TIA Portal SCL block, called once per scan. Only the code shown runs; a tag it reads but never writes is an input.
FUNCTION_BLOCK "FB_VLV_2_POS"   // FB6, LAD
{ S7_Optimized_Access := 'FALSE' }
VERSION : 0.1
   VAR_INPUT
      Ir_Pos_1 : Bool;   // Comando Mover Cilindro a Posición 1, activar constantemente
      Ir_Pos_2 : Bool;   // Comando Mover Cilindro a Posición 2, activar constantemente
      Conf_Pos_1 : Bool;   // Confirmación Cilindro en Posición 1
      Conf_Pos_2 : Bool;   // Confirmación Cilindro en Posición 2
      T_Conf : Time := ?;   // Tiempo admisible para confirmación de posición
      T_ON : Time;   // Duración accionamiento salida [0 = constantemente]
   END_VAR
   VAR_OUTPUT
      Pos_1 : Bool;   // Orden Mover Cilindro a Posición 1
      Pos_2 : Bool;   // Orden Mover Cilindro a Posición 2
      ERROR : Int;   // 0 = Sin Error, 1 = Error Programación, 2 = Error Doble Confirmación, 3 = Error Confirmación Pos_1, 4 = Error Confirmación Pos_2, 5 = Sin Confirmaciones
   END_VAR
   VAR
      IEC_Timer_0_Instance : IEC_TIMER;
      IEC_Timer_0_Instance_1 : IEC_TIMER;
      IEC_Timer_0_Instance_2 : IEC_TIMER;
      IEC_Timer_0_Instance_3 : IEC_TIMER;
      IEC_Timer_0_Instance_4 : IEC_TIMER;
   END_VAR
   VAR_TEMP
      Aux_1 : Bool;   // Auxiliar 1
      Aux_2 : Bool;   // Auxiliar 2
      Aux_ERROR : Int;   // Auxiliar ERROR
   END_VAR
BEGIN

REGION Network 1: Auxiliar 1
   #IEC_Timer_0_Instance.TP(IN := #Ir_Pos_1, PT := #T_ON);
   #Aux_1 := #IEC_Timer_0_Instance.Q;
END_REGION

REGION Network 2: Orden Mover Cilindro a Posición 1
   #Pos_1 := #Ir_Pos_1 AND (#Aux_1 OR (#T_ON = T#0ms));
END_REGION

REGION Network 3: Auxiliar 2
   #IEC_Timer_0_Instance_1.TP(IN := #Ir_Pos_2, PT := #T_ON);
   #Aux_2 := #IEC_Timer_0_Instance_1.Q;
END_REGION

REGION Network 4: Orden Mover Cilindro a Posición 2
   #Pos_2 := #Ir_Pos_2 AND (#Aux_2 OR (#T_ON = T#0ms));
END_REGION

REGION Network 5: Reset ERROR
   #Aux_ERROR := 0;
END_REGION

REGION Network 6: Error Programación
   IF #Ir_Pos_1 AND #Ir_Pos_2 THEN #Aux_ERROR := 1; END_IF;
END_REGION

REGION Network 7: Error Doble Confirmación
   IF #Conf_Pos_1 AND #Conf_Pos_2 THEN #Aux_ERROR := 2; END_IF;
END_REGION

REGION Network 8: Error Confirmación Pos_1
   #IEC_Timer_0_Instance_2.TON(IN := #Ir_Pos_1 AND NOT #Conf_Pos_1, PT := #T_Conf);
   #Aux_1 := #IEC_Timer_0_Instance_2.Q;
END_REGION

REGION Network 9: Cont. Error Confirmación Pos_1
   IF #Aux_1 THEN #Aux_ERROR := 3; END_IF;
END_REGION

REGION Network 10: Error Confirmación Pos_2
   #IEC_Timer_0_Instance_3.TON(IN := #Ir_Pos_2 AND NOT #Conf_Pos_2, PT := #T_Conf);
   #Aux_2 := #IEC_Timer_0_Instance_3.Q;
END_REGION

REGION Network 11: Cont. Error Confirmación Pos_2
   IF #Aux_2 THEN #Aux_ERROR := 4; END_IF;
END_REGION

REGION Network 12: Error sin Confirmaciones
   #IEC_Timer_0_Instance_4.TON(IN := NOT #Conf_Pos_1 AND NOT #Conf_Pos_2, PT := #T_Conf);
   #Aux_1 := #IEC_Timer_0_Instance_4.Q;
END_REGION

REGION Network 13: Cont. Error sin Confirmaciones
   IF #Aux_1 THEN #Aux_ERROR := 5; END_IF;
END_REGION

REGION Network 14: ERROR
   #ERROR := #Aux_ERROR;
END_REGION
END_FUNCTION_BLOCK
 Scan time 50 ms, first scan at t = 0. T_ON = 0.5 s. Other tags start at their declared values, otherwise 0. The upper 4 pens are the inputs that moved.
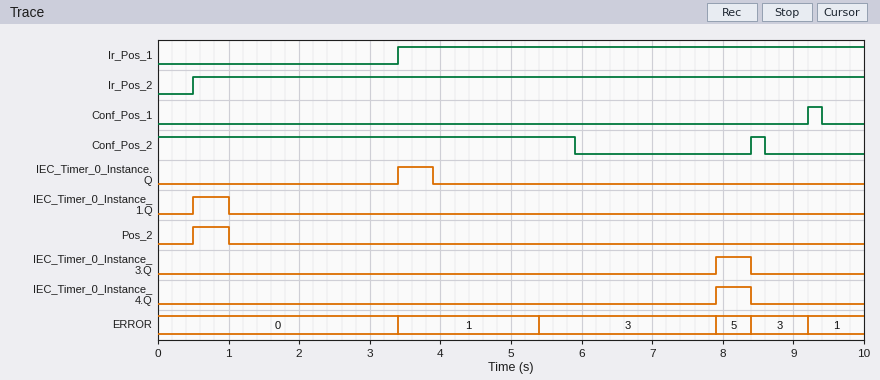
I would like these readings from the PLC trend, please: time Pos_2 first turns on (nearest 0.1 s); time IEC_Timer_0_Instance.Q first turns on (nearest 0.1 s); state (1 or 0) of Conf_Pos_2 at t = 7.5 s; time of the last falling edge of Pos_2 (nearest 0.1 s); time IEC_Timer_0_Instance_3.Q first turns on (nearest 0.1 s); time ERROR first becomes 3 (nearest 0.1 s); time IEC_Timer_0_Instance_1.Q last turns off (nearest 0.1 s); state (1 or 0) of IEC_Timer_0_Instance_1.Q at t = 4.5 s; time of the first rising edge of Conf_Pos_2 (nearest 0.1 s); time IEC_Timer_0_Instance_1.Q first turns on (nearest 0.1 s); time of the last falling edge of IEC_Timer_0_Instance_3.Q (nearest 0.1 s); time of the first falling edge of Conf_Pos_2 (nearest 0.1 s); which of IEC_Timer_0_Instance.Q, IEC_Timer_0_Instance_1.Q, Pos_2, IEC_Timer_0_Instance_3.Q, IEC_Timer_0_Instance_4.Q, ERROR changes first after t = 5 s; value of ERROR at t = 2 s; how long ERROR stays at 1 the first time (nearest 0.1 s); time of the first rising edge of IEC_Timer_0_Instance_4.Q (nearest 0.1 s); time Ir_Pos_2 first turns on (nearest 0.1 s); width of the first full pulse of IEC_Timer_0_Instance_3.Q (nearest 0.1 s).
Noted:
0.5 s
3.4 s
0
1.0 s
7.9 s
5.4 s
1.0 s
0
8.4 s
0.5 s
8.4 s
5.9 s
ERROR
0
2.0 s
7.9 s
0.5 s
0.5 s
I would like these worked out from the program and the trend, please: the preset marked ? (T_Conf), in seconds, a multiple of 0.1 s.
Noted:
2.0 s
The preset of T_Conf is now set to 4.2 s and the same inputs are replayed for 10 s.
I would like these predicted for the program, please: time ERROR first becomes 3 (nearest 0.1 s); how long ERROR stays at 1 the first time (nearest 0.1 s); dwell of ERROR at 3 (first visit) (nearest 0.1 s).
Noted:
7.6 s
4.2 s
1.6 s
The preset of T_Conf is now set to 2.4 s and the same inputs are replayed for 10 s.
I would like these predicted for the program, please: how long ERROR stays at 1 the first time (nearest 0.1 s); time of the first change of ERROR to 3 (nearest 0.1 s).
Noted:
2.4 s
5.8 s
